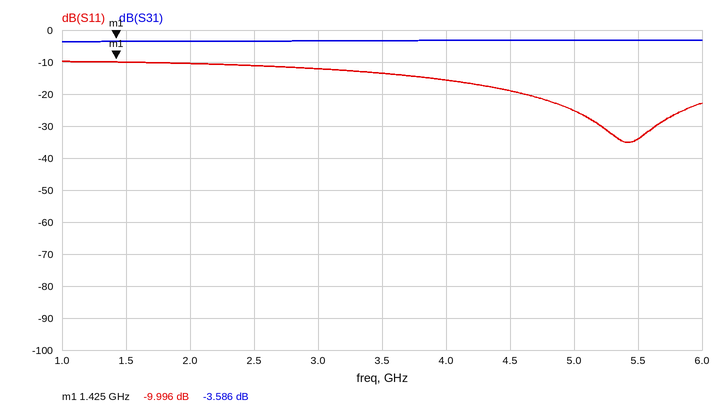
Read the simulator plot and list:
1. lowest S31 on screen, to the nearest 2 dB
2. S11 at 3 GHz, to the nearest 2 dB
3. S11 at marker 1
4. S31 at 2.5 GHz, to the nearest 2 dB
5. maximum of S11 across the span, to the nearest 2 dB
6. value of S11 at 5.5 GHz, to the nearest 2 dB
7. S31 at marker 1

-4 dB
-12 dB
-9.996 dB
-4 dB
-10 dB
-34 dB
-3.586 dB
